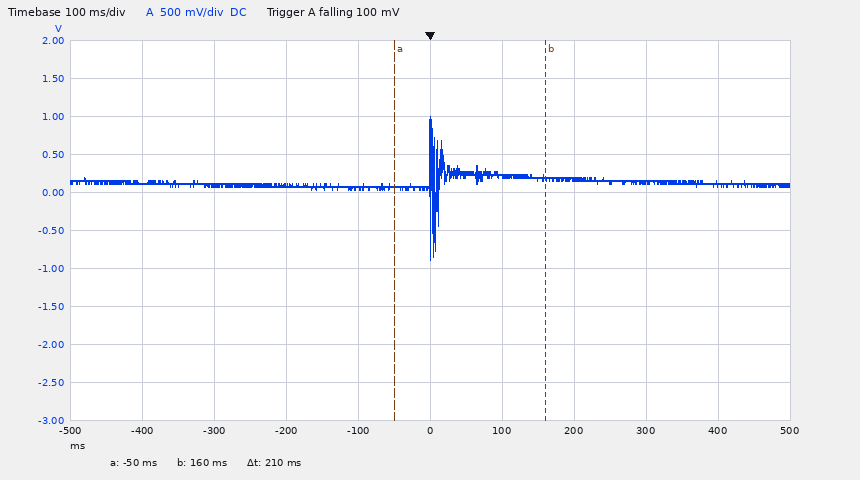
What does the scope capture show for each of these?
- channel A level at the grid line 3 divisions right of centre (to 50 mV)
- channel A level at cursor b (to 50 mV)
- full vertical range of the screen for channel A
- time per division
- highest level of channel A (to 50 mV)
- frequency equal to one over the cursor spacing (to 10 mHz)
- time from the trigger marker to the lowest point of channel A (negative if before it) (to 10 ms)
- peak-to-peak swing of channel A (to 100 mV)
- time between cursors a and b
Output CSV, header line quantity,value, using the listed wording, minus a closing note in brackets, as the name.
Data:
quantity,value
channel A level at the grid line 3 divisions right of centre,150 mV
channel A level at cursor b,200 mV
full vertical range of the screen for channel A,5 V
time per division,100 ms
highest level of channel A,1.00 V
frequency equal to one over the cursor spacing,4.76 Hz
time from the trigger marker to the lowest point of channel A (negative if before it),0 ms
peak-to-peak swing of channel A,1.90 V
time between cursors a and b,210 ms
